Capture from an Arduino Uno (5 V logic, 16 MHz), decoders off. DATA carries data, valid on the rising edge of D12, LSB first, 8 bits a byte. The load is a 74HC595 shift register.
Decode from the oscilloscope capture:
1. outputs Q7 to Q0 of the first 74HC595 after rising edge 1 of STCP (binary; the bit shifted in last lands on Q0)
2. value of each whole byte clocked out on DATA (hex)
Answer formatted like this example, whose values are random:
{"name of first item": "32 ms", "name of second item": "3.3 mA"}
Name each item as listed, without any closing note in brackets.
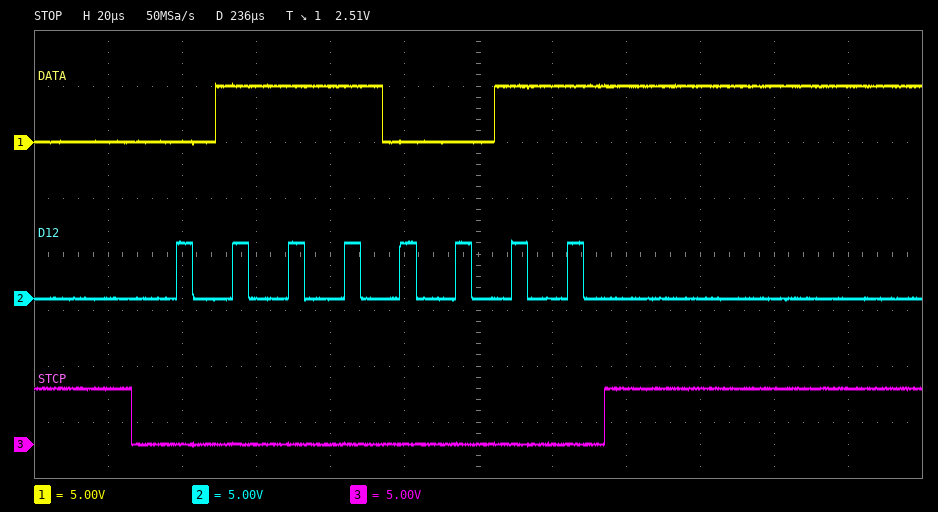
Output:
{"outputs Q7 to Q0 of the first 74HC595 after rising edge 1 of STCP": "01110011", "value of each whole byte clocked out on DATA": "CE"}
